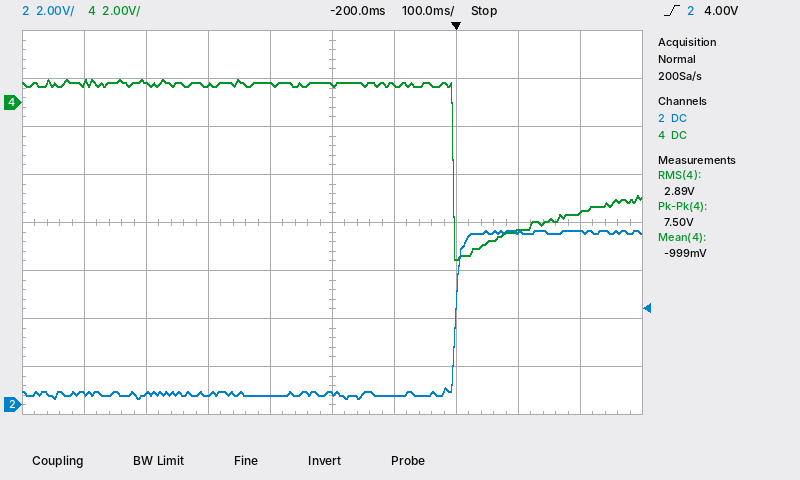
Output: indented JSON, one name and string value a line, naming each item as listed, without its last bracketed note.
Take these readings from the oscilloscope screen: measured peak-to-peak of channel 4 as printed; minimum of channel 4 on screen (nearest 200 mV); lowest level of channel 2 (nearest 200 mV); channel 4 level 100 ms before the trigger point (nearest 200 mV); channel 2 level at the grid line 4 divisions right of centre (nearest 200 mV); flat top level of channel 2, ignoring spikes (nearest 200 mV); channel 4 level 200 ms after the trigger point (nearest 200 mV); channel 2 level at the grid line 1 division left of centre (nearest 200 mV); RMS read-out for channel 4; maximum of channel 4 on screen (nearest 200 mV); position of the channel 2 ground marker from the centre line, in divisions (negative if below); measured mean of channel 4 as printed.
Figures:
{
  "measured peak-to-peak of channel 4 as printed": "7.50 V",
  "minimum of channel 4 on screen": "-6.6 V",
  "lowest level of channel 2": "200 mV",
  "channel 4 level 100 ms before the trigger point": "800 mV",
  "channel 2 level at the grid line 4 divisions right of centre": "7.2 V",
  "flat top level of channel 2, ignoring spikes": "7.2 V",
  "channel 4 level 200 ms after the trigger point": "-4.6 V",
  "channel 2 level at the grid line 1 division left of centre": "400 mV",
  "RMS read-out for channel 4": "2.89 V",
  "maximum of channel 4 on screen": "1.0 V",
  "position of the channel 2 ground marker from the centre line, in divisions": "-3.8 div",
  "measured mean of channel 4 as printed": "-999 mV"
}
